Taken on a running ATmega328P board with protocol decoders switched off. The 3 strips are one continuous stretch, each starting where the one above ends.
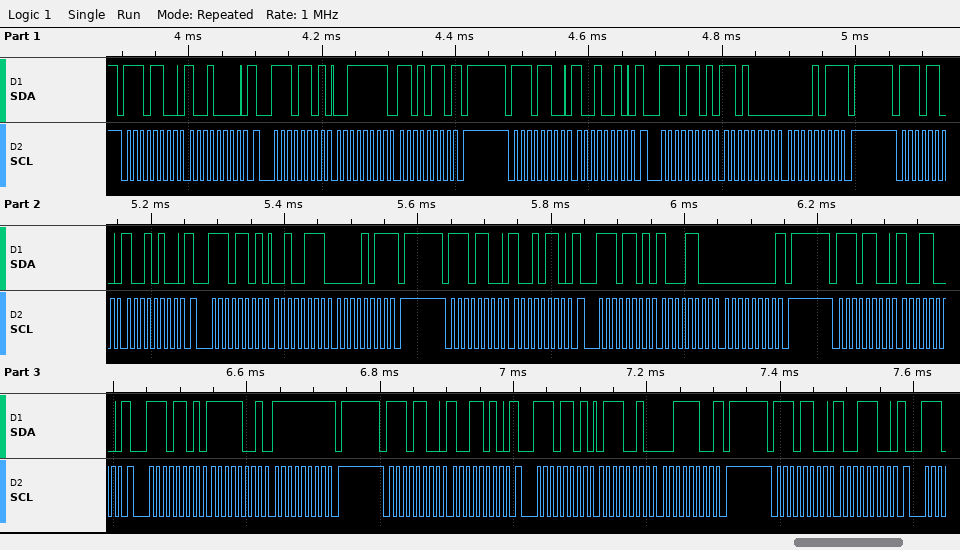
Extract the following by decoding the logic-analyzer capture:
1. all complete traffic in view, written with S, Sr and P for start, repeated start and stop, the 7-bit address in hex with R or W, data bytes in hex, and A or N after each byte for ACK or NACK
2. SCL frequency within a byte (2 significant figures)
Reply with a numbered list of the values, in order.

1. S 76W A 90 A Sr 76R A 3F A D6 N P S 76W A 92 A Sr 76R A D0 A 0B N P S 76W A 94 A Sr 76R A 27 A 0B N P S 76W A 96 A Sr 76R A 8C A 00 N P S 76W A 98 A Sr 76R A F9 A FF N P S 76W A 9A A Sr 76R A 72 A 3C N P S 76W A 9C A
2. 100 kHz
